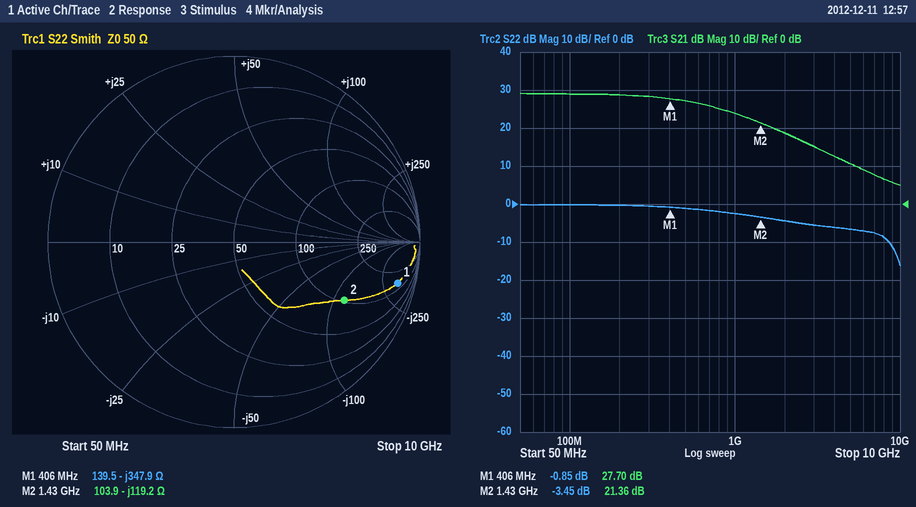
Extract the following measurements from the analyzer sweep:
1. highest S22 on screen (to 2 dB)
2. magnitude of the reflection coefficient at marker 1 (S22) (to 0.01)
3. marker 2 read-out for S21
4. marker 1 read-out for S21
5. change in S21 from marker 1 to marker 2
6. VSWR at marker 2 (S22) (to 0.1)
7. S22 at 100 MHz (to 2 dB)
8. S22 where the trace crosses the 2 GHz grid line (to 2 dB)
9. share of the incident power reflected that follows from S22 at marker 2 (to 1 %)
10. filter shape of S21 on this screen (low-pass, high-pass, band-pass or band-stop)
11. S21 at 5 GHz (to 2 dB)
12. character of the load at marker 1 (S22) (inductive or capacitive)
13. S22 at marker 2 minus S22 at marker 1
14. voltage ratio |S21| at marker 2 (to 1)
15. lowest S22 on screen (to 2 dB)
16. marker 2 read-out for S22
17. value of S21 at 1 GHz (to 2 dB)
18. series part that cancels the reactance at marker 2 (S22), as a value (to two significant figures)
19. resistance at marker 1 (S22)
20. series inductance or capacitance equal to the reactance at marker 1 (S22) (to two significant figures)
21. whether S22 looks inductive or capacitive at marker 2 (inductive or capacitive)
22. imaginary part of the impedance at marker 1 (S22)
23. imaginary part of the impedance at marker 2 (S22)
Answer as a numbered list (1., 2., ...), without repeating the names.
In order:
1. 0 dB
2. 0.91
3. 21.36 dB
4. 27.70 dB
5. -6.34 dB
6. 5.1
7. 0 dB
8. -4 dB
9. 45 %
10. low-pass
11. 10 dB
12. capacitive
13. -2.60 dB
14. 12
15. -16 dB
16. -3.45 dB
17. 24 dB
18. 13 nH
19. 139.5 Ω
20. 1.1 pF
21. capacitive
22. -347.9 Ω
23. -119.2 Ω
